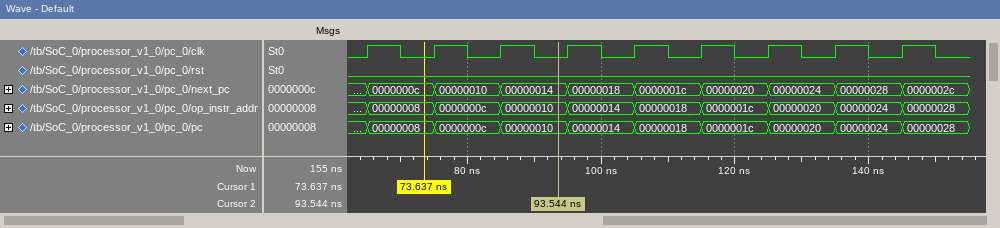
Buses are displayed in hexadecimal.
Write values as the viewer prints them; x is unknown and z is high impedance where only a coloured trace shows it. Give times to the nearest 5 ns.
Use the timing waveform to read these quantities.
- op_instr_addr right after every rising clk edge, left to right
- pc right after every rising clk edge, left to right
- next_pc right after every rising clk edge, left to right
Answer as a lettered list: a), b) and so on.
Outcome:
a) 00000008, 0000000c, 00000010, 00000014, 00000018, 0000001c, 00000020, 00000024, 00000028
b) 00000008, 0000000c, 00000010, 00000014, 00000018, 0000001c, 00000020, 00000024, 00000028
c) 0000000c, 00000010, 00000014, 00000018, 0000001c, 00000020, 00000024, 00000028, 0000002c
